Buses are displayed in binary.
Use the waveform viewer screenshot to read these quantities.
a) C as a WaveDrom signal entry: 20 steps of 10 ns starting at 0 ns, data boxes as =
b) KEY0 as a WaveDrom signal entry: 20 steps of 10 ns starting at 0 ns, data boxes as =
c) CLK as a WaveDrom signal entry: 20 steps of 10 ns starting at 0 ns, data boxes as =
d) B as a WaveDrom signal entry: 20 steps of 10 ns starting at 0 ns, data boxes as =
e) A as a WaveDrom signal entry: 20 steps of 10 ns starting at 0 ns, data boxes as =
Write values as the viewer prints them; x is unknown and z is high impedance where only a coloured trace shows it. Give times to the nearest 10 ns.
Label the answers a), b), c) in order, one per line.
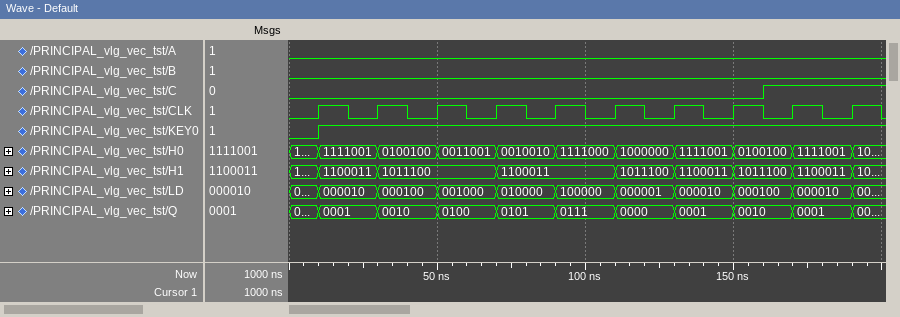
a) {name: 'C', wave: '0...............1...'}
b) {name: 'KEY0', wave: '01..................'}
c) {name: 'CLK', wave: '01010101010101010101'}
d) {name: 'B', wave: '0...................'}
e) {name: 'A', wave: '0...................'}
